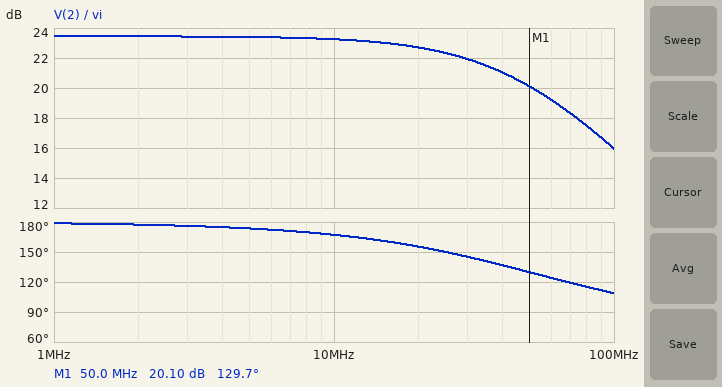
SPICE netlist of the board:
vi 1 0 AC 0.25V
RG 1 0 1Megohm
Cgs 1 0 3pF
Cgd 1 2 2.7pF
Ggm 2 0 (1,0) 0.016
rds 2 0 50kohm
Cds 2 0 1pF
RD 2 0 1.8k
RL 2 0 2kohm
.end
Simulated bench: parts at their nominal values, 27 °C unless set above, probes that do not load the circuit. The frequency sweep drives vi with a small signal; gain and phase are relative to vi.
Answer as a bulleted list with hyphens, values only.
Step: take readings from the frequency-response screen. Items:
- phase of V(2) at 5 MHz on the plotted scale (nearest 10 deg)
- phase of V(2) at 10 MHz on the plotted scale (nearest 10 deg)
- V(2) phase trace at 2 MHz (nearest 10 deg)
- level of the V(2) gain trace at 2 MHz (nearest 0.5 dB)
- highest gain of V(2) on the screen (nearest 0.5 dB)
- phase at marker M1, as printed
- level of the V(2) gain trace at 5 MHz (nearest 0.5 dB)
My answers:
- 170 deg
- 170 deg
- 180 deg
- 23.5 dB
- 23.5 dB
- 129.7 deg
- 23.5 dB
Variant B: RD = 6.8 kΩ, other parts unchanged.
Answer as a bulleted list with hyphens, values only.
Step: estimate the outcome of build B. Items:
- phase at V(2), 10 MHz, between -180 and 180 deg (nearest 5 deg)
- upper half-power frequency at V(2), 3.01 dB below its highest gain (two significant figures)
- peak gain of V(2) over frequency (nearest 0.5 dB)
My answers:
- 160 deg
- 29 MHz
- 27.5 dB
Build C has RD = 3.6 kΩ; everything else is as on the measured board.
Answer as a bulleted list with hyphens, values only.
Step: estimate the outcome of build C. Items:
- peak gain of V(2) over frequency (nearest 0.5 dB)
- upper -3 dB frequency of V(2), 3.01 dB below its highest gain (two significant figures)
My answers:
- 26.0 dB
- 34 MHz
